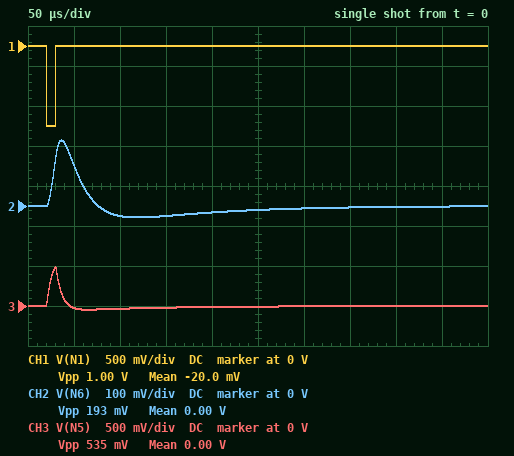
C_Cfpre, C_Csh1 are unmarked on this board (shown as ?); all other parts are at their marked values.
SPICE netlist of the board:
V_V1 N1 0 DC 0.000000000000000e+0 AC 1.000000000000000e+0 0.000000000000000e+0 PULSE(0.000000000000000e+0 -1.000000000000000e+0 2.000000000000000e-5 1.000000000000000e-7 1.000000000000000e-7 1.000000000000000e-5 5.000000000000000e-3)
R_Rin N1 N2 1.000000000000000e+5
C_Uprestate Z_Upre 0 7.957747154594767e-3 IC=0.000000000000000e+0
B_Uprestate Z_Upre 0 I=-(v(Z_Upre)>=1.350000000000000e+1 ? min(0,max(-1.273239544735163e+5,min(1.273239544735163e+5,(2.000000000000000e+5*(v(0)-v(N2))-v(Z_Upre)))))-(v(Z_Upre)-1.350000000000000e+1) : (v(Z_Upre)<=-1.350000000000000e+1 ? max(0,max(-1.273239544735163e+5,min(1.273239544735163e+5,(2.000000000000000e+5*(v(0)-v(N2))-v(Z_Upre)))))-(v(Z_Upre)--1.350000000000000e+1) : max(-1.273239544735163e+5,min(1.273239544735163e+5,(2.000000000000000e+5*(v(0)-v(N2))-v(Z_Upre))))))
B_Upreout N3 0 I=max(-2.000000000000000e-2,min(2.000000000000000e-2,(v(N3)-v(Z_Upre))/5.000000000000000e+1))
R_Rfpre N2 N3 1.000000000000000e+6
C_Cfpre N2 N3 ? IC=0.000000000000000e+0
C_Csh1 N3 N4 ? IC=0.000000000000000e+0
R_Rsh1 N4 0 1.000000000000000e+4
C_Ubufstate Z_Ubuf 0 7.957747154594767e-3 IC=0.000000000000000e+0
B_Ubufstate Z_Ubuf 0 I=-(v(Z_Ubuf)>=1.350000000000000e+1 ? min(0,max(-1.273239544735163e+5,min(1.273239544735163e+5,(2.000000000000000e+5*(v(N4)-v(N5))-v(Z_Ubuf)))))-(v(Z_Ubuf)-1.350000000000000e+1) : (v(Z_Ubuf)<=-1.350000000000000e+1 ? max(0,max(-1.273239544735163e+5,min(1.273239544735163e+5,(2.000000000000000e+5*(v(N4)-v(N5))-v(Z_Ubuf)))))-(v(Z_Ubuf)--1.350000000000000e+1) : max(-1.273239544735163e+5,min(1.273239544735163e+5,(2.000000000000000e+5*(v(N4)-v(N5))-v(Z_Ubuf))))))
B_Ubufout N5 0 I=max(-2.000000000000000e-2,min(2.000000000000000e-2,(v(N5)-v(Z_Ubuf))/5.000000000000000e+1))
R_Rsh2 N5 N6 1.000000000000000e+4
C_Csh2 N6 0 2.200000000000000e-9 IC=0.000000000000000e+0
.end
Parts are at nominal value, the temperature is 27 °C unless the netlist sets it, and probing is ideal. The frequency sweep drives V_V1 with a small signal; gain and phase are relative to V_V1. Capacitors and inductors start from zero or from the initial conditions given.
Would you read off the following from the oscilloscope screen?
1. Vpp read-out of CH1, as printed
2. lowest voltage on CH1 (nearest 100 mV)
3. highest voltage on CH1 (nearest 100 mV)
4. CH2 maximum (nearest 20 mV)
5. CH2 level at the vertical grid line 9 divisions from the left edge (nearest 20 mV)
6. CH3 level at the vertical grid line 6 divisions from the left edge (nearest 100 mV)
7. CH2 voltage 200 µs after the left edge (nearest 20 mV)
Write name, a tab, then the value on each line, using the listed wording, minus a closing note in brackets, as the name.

Vpp read-out of CH1, as printed	1.00 V
lowest voltage on CH1	-1.0 V
highest voltage on CH1	0 V
CH2 maximum	160 mV
CH2 level at the vertical grid line 9 divisions from the left edge	0 V
CH3 level at the vertical grid line 6 divisions from the left edge	0 V
CH2 voltage 200 µs after the left edge	-20 mV
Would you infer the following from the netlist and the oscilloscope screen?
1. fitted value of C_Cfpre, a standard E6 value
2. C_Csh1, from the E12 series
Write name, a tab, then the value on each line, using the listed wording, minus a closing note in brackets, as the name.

fitted value of C_Cfpre, a standard E6 value	100 pF
C_Csh1, from the E12 series	680 pF
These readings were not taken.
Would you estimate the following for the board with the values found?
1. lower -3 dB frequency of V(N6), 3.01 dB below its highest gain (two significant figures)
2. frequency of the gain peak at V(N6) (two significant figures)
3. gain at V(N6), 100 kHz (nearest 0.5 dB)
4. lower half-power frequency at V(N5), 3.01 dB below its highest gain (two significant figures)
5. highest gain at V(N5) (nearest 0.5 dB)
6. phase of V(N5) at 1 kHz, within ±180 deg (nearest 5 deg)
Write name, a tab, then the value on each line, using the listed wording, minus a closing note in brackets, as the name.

lower -3 dB frequency of V(N6), 3.01 dB below its highest gain	1.1 kHz
frequency of the gain peak at V(N6)	3.3 kHz
gain at V(N6), 100 kHz	-39.0 dB
lower half-power frequency at V(N5), 3.01 dB below its highest gain	1.4 kHz
highest gain at V(N5)	-4.0 dB
phase of V(N5) at 1 kHz, within ±180 deg	-125 deg
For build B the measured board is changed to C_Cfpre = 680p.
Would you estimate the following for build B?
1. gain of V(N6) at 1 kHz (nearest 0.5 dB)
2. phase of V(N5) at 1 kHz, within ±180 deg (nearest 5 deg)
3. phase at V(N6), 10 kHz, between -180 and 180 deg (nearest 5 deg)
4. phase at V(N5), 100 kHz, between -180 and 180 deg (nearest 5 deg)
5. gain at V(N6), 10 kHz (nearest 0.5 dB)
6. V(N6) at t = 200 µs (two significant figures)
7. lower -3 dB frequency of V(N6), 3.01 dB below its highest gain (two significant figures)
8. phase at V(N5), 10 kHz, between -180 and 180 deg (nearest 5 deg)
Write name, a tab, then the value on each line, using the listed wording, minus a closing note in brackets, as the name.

gain of V(N6) at 1 kHz	-20.5 dB
phase of V(N5) at 1 kHz, within ±180 deg	-170 deg
phase at V(N6), 10 kHz, between -180 and 180 deg	105 deg
phase at V(N5), 100 kHz, between -180 and 180 deg	100 deg
gain at V(N6), 10 kHz	-25.5 dB
V(N6) at t = 200 µs	-1.2 mV
lower -3 dB frequency of V(N6), 3.01 dB below its highest gain	220 Hz
phase at V(N5), 10 kHz, between -180 and 180 deg	160 deg
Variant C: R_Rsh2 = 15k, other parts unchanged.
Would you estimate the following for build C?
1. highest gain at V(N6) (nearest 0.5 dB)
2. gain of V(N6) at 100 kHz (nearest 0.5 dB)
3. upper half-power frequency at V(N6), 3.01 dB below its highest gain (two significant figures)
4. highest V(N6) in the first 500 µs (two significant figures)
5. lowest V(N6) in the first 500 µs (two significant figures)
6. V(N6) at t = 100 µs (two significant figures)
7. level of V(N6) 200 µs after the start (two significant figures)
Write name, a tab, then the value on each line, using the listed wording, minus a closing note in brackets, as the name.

highest gain at V(N6)	-6.0 dB
gain of V(N6) at 100 kHz	-42.5 dB
upper half-power frequency at V(N6), 3.01 dB below its highest gain	7.0 kHz
highest V(N6) in the first 500 µs	120 mV
lowest V(N6) in the first 500 µs	-23 mV
V(N6) at t = 100 µs	-11 mV
level of V(N6) 200 µs after the start	-17 mV
